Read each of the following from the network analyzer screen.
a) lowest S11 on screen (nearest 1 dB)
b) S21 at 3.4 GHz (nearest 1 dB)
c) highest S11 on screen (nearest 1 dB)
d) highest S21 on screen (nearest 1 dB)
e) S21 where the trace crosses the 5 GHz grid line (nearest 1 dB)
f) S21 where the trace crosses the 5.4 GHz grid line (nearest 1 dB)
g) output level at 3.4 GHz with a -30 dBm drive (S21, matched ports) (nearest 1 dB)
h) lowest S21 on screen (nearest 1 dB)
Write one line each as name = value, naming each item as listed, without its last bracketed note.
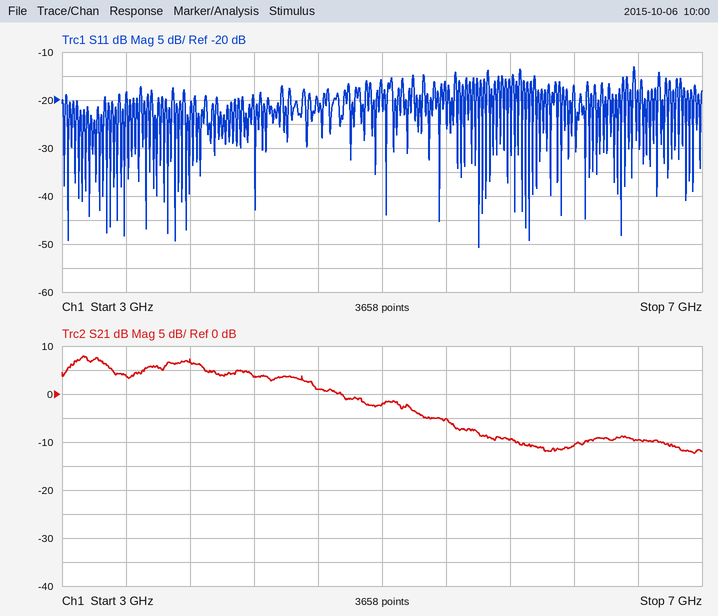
lowest S11 on screen = -51 dB
S21 at 3.4 GHz = 4 dB
highest S11 on screen = -13 dB
highest S21 on screen = 8 dB
S21 where the trace crosses the 5 GHz grid line = -2 dB
S21 where the trace crosses the 5.4 GHz grid line = -5 dB
output level at 3.4 GHz with a -30 dBm drive (S21, matched ports) = -26 dBm
lowest S21 on screen = -12 dB
